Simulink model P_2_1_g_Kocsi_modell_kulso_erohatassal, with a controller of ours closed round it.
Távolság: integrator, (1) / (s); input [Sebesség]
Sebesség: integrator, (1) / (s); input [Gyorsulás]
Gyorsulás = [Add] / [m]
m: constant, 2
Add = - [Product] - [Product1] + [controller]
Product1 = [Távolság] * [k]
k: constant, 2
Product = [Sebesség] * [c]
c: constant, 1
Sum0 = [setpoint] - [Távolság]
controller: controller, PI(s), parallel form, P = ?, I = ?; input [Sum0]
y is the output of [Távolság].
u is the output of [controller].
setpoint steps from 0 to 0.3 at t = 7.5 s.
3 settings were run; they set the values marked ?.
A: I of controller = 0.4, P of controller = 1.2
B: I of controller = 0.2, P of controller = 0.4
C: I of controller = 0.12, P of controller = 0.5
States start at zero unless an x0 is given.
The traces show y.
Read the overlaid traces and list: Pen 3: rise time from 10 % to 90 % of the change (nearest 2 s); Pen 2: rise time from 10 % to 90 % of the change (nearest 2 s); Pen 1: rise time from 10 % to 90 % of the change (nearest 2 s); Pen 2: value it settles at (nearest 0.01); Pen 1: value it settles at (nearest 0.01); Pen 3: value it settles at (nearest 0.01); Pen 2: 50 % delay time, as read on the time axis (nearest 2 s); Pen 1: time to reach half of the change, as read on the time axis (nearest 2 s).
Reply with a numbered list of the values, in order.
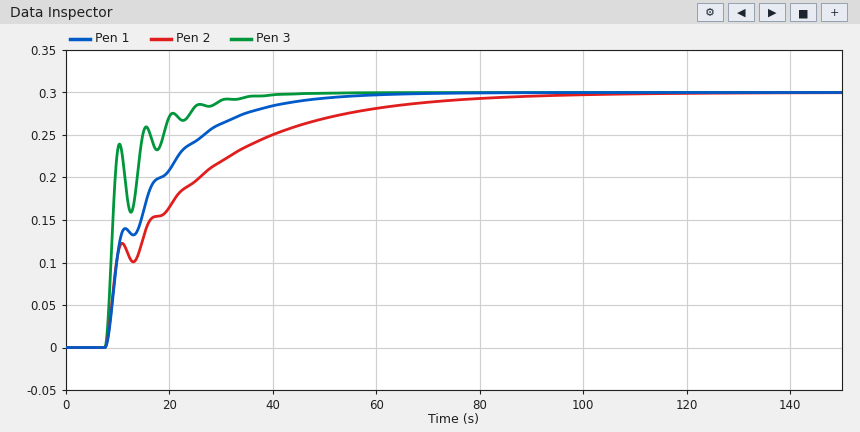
1. 12 s
2. 42 s
3. 24 s
4. 0.30
5. 0.30
6. 0.30
7. 16 s
8. 14 s
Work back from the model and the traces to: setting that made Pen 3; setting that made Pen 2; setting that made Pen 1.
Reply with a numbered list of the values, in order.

1. A
2. C
3. B
